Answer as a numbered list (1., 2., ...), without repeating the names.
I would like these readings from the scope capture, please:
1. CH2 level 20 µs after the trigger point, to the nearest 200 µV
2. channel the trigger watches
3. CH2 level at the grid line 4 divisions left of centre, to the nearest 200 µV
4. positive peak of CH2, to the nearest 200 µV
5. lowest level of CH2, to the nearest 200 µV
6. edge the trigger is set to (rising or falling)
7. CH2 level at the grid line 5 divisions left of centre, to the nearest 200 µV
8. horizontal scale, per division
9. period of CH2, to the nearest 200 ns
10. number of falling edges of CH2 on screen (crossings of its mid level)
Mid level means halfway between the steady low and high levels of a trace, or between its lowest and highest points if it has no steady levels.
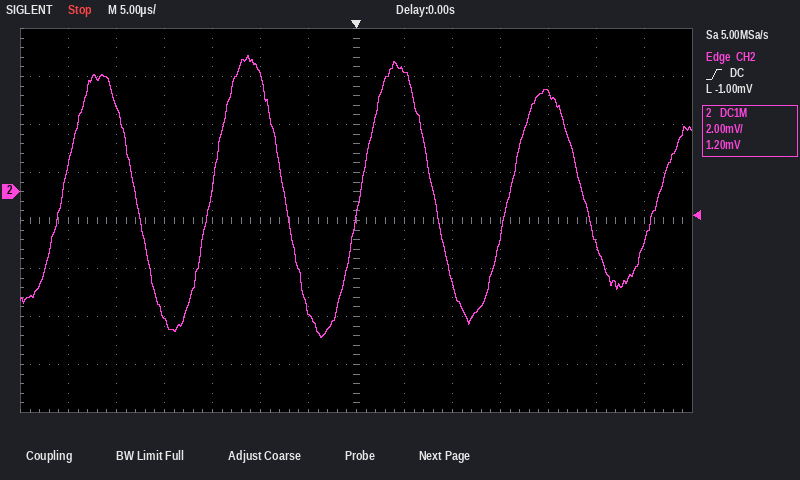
1. 4.2 mV
2. CH2
3. -5.2 mV
4. 5.6 mV
5. -6.0 mV
6. rising
7. 3.6 mV
8. 5 µs
9. 15.6 µs
10. 4
